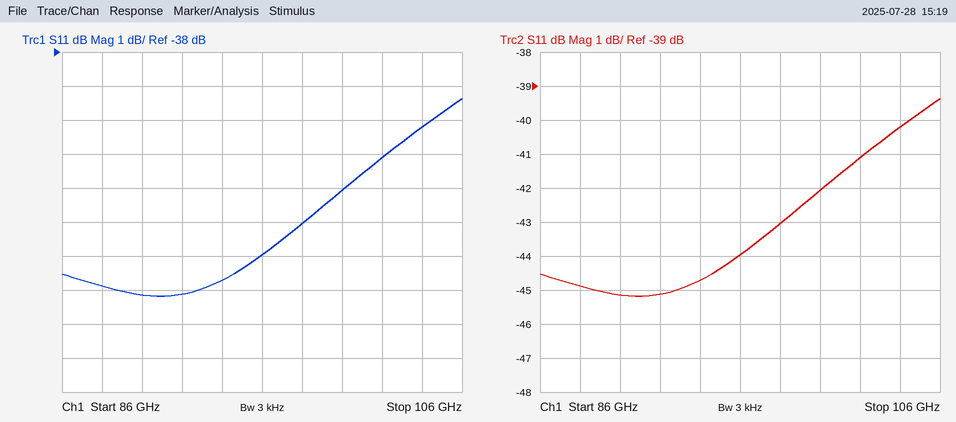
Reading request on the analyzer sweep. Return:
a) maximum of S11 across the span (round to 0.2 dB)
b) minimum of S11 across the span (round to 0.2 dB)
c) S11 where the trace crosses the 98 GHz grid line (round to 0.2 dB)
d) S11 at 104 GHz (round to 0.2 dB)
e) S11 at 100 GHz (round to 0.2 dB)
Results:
-39.4 dB
-45.2 dB
-43.0 dB
-40.2 dB
-42.0 dB
